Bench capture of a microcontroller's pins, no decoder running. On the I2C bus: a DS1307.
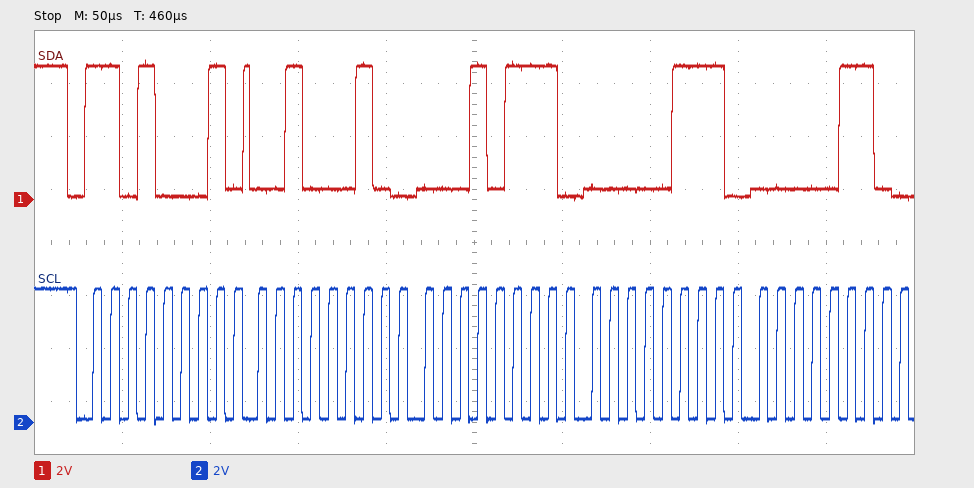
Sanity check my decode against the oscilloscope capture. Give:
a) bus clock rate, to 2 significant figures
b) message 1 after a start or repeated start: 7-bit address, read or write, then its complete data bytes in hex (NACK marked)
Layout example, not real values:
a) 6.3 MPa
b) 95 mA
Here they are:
a) 100 kHz
b) 0x68 read: 22 17 07 06
